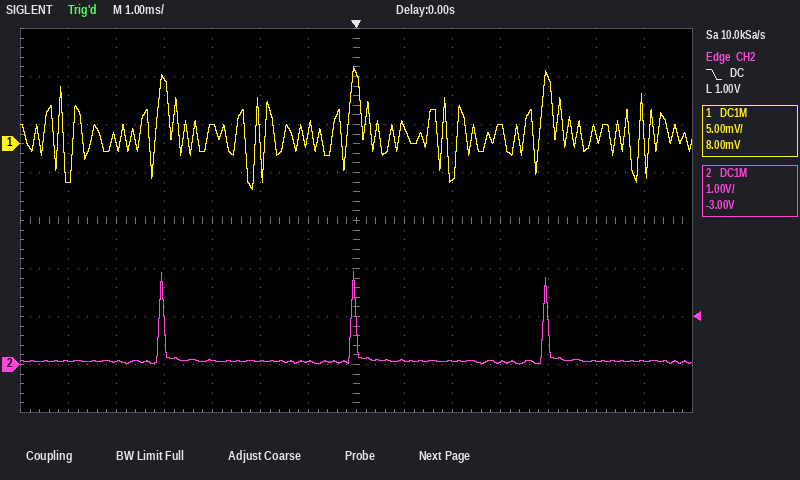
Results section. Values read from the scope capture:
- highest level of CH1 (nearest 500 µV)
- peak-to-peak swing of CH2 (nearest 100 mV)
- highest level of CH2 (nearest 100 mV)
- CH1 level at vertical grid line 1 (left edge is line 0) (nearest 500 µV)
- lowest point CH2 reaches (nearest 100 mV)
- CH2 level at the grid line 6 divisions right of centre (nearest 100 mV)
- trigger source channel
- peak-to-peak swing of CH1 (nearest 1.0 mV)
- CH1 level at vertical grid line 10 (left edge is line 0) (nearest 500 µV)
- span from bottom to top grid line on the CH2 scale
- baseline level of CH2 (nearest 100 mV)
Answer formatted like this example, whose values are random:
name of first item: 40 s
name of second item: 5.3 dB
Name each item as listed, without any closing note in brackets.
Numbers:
highest level of CH1: 8.0 mV
peak-to-peak swing of CH2: 1.9 V
highest level of CH2: 1.9 V
CH1 level at vertical grid line 1 (left edge is line 0): -4.0 mV
lowest point CH2 reaches: 0.0 V
CH2 level at the grid line 6 divisions right of centre: 100 mV
trigger source channel: CH2
peak-to-peak swing of CH1: 13.0 mV
CH1 level at vertical grid line 10 (left edge is line 0): 2.0 mV
span from bottom to top grid line on the CH2 scale: 8 V
baseline level of CH2: 100 mV
